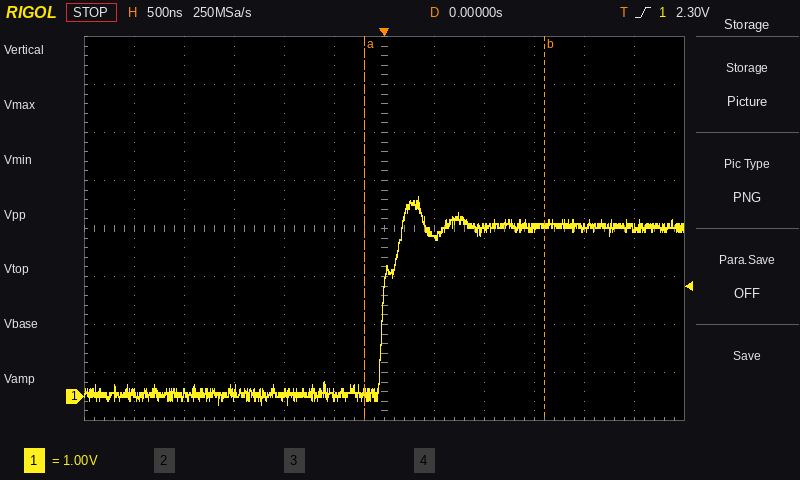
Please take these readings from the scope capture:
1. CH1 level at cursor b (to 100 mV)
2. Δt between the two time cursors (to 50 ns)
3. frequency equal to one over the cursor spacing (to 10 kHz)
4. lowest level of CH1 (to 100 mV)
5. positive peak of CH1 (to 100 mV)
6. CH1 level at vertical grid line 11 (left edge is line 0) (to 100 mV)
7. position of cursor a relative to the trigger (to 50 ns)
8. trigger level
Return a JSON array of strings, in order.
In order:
["3.6 V", "1.80 µs", "560 kHz", "-200 mV", "4.2 V", "3.5 V", "-200 ns", "2.30 V"]
